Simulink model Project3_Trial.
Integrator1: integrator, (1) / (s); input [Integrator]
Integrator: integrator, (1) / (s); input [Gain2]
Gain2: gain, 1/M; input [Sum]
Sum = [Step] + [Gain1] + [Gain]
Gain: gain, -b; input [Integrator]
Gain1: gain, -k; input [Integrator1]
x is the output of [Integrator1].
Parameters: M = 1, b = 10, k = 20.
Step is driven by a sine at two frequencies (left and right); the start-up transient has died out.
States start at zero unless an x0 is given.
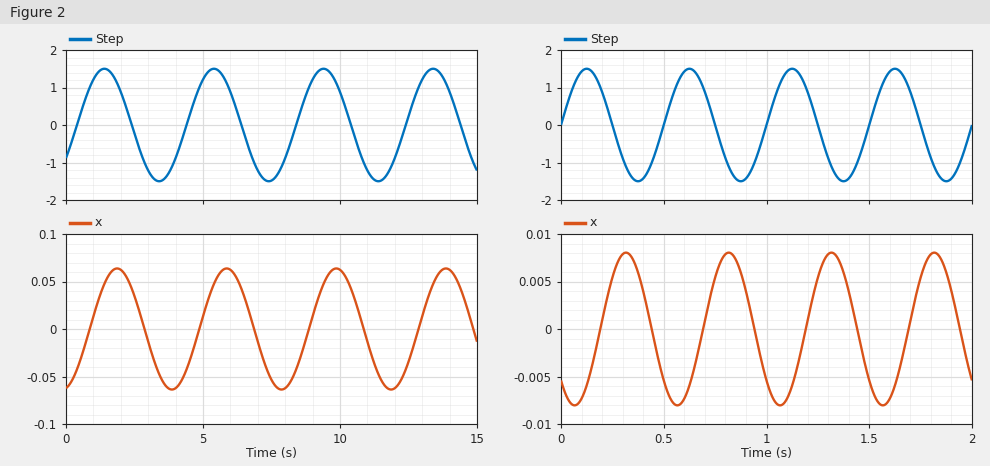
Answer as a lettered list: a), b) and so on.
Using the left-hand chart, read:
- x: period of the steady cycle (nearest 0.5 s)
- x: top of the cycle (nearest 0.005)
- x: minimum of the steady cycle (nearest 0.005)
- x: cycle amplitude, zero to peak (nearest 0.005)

a) 4.0 s
b) 0.065
c) -0.065
d) 0.065
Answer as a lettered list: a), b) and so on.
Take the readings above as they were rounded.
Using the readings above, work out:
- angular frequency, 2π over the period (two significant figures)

a) 1.6 rad/s
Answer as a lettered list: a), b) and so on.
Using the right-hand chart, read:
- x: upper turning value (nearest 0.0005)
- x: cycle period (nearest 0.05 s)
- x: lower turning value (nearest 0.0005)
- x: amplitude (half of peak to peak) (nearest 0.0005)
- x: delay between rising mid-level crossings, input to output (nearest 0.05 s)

a) 0.0080
b) 0.50 s
c) -0.0080
d) 0.0080
e) 0.20 s
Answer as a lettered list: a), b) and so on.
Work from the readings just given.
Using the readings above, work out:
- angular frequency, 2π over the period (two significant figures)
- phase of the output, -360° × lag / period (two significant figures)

a) 13 rad/s
b) -140°
